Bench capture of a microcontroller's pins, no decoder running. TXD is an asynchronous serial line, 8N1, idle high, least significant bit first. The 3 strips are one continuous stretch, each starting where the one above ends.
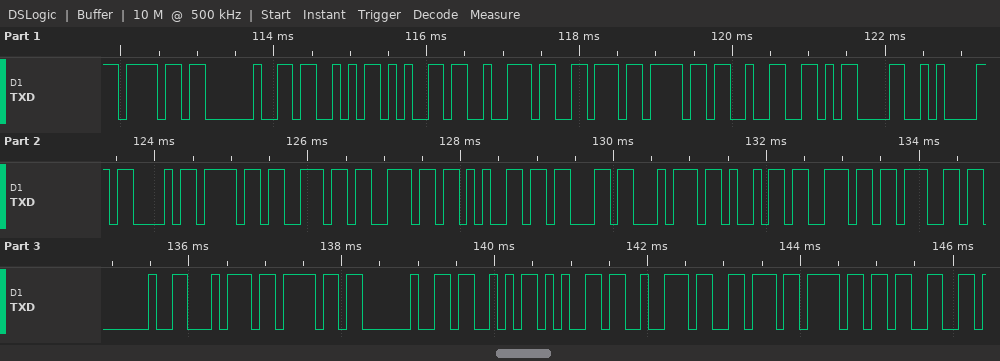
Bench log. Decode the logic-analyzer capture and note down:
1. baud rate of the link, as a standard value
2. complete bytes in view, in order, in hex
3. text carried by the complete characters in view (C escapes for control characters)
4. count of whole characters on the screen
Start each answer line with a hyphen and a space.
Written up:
- 9600 baud
- 6F 20 53 65 72 76 6F 32 0D 0A 43 6F 6E 6E 65 63 74 69 6E 67 20 74 6F 20 53 65 72 76 6F 33
- "o Servo2\r\nConnecting to Servo3"
- 30
